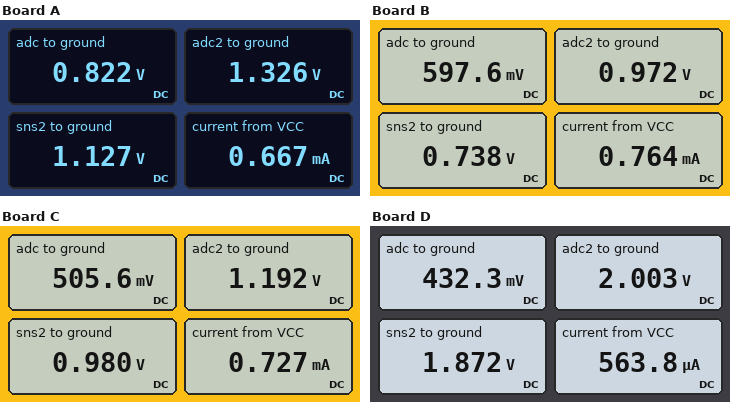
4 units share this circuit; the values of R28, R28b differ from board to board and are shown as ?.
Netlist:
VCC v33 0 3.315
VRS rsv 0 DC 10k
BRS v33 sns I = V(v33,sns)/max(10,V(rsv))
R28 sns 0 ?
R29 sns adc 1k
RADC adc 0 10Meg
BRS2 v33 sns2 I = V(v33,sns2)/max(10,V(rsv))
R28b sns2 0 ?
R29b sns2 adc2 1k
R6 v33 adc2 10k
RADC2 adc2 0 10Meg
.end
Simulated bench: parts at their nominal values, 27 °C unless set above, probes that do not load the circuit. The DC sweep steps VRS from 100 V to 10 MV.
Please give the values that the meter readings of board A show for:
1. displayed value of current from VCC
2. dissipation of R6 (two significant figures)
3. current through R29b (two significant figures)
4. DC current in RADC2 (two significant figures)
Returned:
0.667 mA
400 µW
200 µA
130 nA
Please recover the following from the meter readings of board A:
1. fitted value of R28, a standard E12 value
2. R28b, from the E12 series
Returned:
3.3 kΩ
2.7 kΩ
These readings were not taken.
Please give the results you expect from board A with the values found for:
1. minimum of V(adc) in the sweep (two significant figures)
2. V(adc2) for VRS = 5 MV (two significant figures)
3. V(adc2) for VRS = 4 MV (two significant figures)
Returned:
1.1 mV
900 mV
900 mV
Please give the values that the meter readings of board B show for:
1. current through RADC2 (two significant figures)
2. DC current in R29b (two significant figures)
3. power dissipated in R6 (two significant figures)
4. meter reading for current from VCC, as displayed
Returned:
97 nA
230 µA
550 µW
0.764 mA
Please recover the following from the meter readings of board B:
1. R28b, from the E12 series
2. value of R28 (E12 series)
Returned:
1.5 kΩ
2.2 kΩ
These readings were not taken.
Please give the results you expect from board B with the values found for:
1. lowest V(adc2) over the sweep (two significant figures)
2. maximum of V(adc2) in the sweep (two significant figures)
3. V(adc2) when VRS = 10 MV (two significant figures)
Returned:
660 mV
3.1 V
660 mV
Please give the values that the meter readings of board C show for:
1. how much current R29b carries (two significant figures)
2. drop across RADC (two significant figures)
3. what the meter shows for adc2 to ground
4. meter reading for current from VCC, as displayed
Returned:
210 µA
510 mV
1.192 V
0.727 mA
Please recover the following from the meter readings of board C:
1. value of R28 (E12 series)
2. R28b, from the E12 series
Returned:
1.8 kΩ
2.2 kΩ
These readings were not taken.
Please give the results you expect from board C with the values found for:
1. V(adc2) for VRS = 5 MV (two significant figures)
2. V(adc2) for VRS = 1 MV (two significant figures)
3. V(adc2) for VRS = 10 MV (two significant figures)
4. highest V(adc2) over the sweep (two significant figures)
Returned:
800 mV
810 mV
800 mV
3.2 V
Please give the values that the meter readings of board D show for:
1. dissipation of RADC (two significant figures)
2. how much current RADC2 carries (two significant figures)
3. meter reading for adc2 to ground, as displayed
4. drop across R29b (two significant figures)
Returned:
19 nW
200 nA
2.003 V
130 mV
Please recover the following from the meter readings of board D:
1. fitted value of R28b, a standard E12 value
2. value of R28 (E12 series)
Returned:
6.8 kΩ
1.5 kΩ
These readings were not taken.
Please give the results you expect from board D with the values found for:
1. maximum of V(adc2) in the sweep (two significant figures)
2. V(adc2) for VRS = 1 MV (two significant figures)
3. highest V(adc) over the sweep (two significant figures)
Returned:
3.3 V
1.5 V
3.1 V
